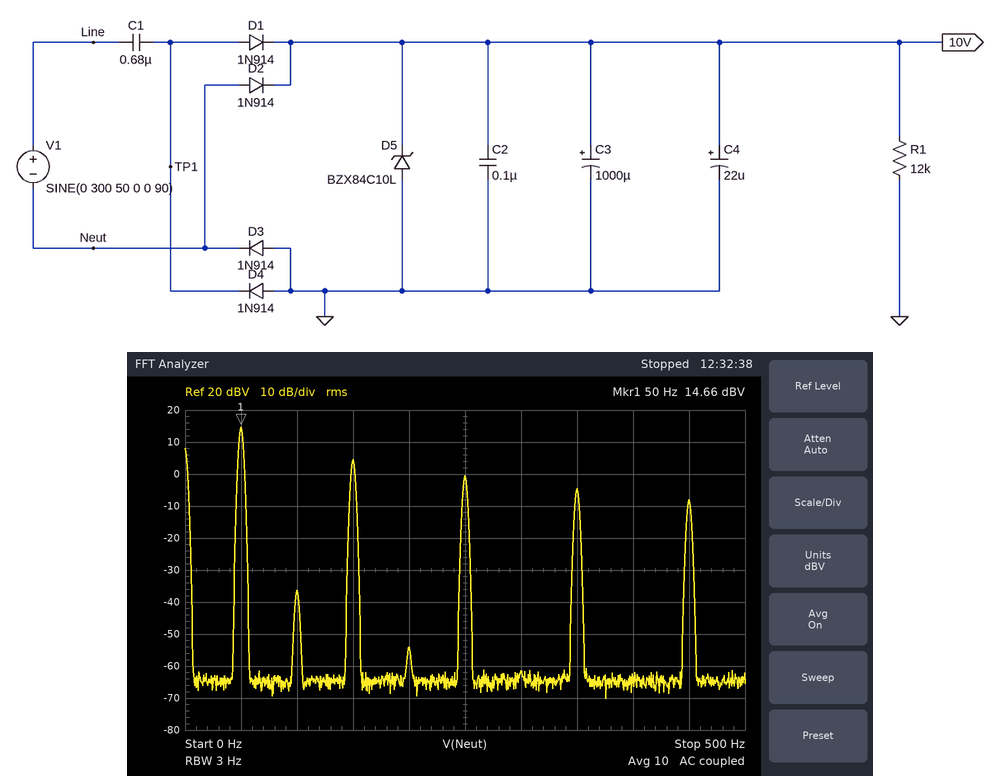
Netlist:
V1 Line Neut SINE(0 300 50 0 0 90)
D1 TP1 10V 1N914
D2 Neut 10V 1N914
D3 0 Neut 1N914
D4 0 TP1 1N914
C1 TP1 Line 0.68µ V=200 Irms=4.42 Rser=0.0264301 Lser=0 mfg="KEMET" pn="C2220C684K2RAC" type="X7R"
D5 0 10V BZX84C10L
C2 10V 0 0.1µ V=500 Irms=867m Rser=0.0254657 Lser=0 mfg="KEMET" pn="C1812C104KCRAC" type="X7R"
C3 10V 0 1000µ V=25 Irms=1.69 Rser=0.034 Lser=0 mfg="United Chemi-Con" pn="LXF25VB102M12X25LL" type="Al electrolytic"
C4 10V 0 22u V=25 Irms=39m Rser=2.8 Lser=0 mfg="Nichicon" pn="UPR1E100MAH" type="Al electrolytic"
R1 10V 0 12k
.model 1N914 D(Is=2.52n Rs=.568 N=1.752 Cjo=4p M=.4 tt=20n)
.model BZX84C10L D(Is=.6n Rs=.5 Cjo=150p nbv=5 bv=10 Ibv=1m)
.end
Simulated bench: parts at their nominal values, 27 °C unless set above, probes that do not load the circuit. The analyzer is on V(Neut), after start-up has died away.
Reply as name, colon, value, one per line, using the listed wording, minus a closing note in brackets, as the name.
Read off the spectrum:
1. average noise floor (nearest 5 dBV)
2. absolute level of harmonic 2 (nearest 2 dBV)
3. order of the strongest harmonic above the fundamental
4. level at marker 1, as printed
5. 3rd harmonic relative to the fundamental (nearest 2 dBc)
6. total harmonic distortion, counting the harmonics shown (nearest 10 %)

average noise floor: -65 dBV
absolute level of harmonic 2: -36 dBV
order of the strongest harmonic above the fundamental: 3
level at marker 1, as printed: 14.66 dBV
3rd harmonic relative to the fundamental: -10 dBc
total harmonic distortion, counting the harmonics shown: 40 %
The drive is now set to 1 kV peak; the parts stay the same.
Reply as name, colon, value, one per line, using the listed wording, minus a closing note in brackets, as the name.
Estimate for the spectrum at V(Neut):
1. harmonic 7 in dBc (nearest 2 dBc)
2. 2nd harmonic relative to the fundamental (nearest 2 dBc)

harmonic 7 in dBc: -18 dBc
2nd harmonic relative to the fundamental: -44 dBc
